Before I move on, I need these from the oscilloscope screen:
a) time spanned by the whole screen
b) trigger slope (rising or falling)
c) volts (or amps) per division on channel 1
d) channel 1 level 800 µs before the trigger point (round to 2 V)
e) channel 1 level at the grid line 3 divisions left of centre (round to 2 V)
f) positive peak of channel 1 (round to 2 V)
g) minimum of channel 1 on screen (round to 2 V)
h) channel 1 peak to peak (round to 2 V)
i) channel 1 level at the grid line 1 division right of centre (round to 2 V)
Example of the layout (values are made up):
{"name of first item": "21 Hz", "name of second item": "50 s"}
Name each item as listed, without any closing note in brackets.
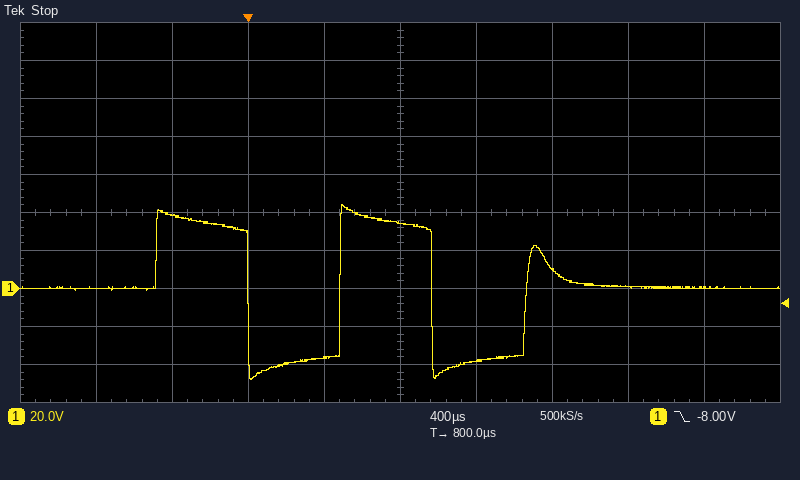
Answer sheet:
{"time spanned by the whole screen": "4 ms", "trigger slope": "falling", "volts (or amps) per division on channel 1": "20 V", "channel 1 level 800 µs before the trigger point": "0 V", "channel 1 level at the grid line 3 divisions left of centre": "38 V", "positive peak of channel 1": "44 V", "minimum of channel 1 on screen": "-48 V", "channel 1 peak to peak": "92 V", "channel 1 level at the grid line 1 division right of centre": "-38 V"}
